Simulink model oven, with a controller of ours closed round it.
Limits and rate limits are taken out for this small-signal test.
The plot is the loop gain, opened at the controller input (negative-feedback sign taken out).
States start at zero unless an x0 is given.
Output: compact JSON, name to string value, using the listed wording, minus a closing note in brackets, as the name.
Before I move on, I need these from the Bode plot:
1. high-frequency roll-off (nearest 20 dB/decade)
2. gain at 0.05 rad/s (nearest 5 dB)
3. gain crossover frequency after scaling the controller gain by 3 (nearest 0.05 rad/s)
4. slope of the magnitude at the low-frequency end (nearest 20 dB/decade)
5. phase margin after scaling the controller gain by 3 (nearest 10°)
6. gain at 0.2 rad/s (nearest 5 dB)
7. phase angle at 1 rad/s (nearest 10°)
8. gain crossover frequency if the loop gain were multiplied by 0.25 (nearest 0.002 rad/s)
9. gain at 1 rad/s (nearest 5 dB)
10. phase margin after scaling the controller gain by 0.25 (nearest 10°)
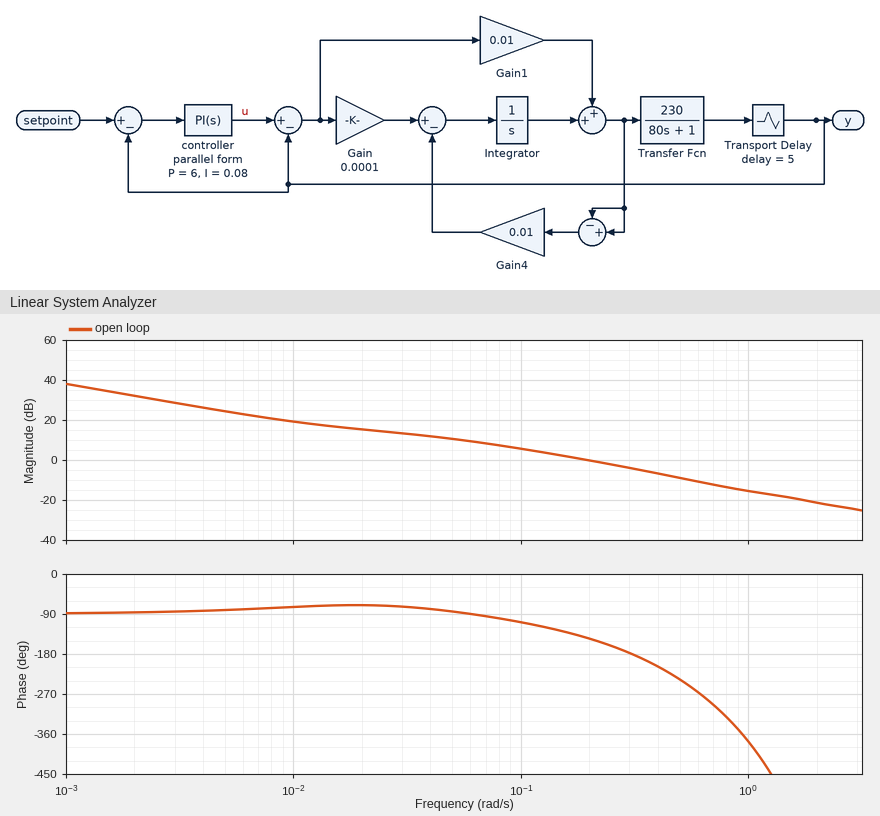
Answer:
{"high-frequency roll-off": "-20 dB/decade", "gain at 0.05 rad/s": "10 dB", "gain crossover frequency after scaling the controller gain by 3": "0.55 rad/s", "slope of the magnitude at the low-frequency end": "-20 dB/decade", "phase margin after scaling the controller gain by 3": "-70°", "gain at 0.2 rad/s": "0 dB", "phase angle at 1 rad/s": "-380°", "gain crossover frequency if the loop gain were multiplied by 0.25": "0.038 rad/s", "gain at 1 rad/s": "-15 dB", "phase margin after scaling the controller gain by 0.25": "100°"}
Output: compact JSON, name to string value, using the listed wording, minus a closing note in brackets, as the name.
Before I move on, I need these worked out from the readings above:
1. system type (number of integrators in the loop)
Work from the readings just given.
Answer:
{"system type": "1"}
